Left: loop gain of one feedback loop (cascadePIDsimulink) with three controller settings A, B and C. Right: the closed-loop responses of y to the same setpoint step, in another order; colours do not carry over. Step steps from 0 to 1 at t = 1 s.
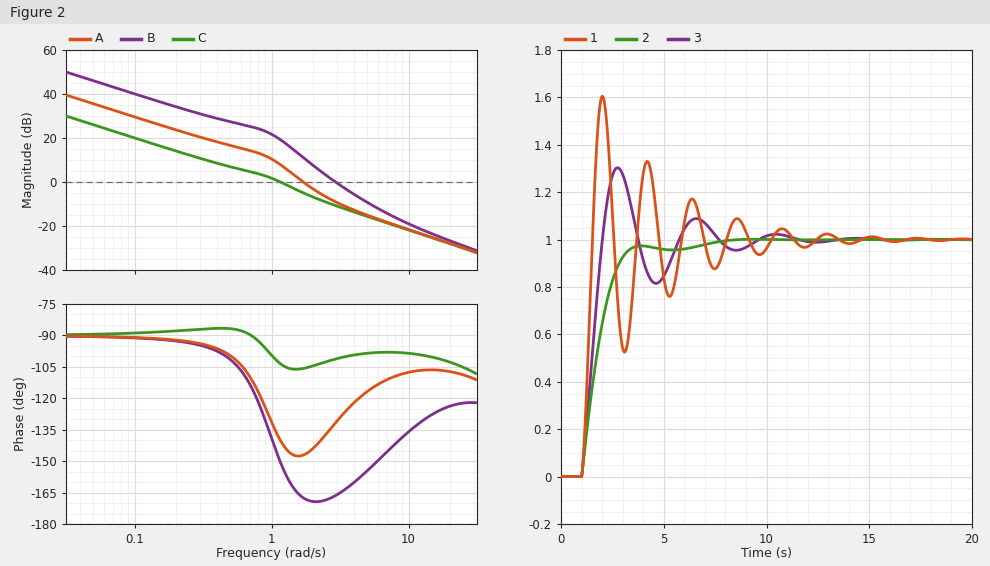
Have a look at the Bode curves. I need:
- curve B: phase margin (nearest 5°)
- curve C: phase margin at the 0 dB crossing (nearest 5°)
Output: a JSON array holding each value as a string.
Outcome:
["15°", "75°"]
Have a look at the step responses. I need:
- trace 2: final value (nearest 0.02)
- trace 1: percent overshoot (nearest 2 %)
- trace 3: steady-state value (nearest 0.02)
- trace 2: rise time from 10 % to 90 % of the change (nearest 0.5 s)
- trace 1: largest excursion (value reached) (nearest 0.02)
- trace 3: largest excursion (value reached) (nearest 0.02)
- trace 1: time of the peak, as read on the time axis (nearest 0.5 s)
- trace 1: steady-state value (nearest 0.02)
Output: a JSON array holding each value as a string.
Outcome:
["1.00", "60 %", "1.00", "1.5 s", "1.60", "1.30", "2.0 s", "1.00"]
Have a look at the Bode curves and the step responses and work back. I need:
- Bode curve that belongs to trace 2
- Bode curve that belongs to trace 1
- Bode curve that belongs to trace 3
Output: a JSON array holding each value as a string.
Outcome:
["C", "B", "A"]
